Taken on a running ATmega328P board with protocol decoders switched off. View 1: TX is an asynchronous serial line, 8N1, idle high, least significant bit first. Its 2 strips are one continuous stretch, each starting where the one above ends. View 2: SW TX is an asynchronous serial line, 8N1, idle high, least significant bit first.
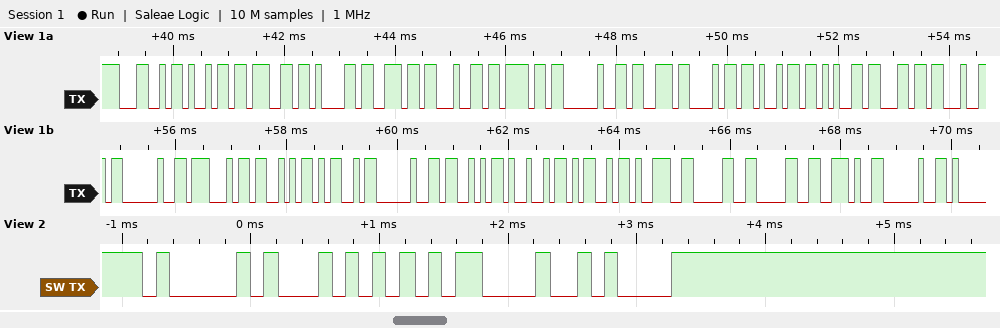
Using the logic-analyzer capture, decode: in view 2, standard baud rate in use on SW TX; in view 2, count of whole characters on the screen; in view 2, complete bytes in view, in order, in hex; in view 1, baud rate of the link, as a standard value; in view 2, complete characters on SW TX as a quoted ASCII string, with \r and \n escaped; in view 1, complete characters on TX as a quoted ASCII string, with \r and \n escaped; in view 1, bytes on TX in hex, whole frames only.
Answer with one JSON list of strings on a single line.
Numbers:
["9600 baud", "4", "41 54 0D 0A", "9600 baud", "\"AT\\r\\n\"", "\"Ligando shield GSM SIM900. \"", "0x4C 0x69 0x67 0x61 0x6E 0x64 0x6F 0x20 0x73 0x68 0x69 0x65 0x6C 0x64 0x20 0x47 0x53 0x4D 0x20 0x53 0x49 0x4D 0x39 0x30 0x30 0x2E 0x20"]
